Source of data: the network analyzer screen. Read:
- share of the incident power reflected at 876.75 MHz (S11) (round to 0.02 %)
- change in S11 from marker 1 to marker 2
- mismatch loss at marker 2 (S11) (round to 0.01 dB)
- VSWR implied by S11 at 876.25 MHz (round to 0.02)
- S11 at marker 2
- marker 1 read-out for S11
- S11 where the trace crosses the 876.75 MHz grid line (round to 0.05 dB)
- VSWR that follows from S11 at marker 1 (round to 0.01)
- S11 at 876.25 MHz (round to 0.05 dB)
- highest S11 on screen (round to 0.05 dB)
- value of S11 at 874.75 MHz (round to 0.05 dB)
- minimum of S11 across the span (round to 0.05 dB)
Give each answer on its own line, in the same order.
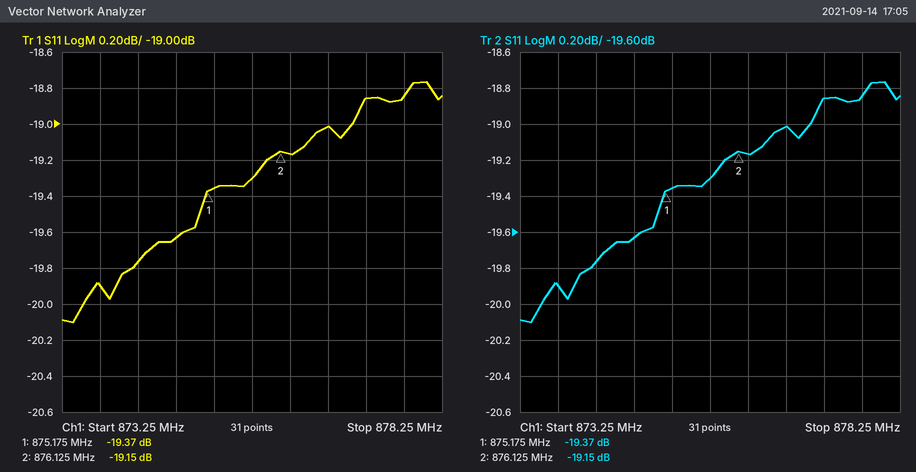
1.26 %
0.22 dB
0.05 dB
1.24
-19.15 dB
-19.37 dB
-19.00 dB
1.24
-19.15 dB
-18.75 dB
-19.65 dB
-20.10 dB
